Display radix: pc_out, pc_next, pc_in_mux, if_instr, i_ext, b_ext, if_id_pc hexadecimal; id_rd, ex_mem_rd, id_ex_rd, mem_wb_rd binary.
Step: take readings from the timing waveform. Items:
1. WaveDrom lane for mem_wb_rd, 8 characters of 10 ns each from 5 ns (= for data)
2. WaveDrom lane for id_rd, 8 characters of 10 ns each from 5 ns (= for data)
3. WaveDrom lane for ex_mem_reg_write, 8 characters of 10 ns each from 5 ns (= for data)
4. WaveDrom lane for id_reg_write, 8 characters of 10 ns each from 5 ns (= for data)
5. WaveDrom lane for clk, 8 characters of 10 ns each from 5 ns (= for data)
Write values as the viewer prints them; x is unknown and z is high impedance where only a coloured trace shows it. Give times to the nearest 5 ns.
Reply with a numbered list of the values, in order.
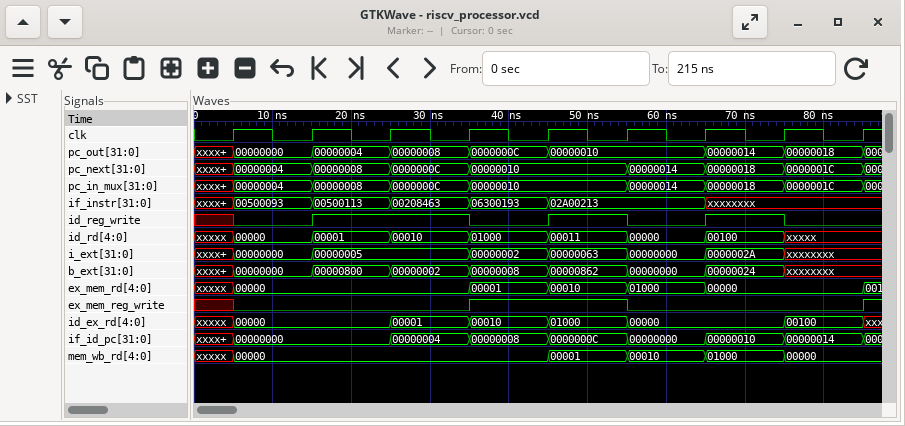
1. {name: 'mem_wb_rd', wave: '=...====', data: '00000 00001 00010 01000 00000'}
2. {name: 'id_rd', wave: '=======x', data: '00000 00001 00010 01000 00011 00000 00100'}
3. {name: 'ex_mem_reg_write', wave: '0..1.0..'}
4. {name: 'id_reg_write', wave: '01.01010'}
5. {name: 'clk', wave: 'p.......'}
